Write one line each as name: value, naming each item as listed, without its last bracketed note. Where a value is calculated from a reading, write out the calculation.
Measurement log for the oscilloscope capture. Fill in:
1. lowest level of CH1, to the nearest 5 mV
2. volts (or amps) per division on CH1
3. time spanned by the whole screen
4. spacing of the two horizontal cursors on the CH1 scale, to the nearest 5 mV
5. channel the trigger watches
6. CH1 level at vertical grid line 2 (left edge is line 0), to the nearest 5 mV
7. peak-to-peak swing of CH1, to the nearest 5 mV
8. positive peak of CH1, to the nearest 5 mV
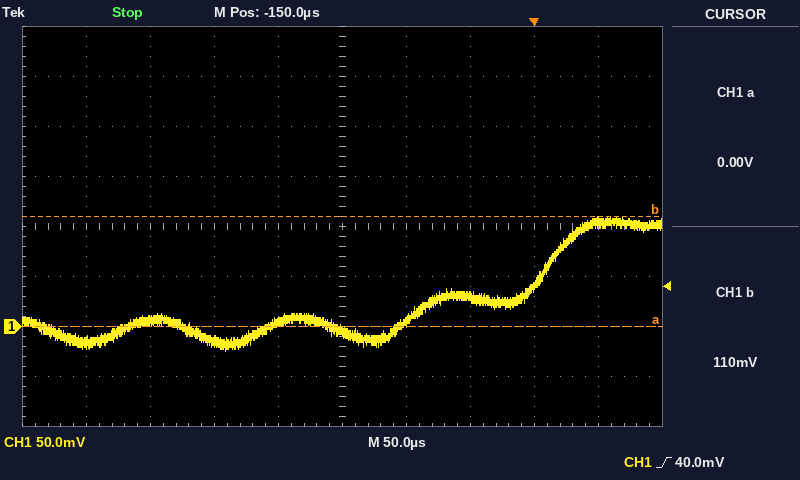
lowest level of CH1, to the nearest 5 mV: -25 mV
volts (or amps) per division on CH1: 50 mV
time spanned by the whole screen: 500 µs
spacing of the two horizontal cursors on the CH1 scale, to the nearest 5 mV: 110 mV
channel the trigger watches: CH1
CH1 level at vertical grid line 2 (left edge is line 0), to the nearest 5 mV: 5 mV
peak-to-peak swing of CH1, to the nearest 5 mV: 110 mV − (-25 mV) = 135 mV
positive peak of CH1, to the nearest 5 mV: 110 mV
